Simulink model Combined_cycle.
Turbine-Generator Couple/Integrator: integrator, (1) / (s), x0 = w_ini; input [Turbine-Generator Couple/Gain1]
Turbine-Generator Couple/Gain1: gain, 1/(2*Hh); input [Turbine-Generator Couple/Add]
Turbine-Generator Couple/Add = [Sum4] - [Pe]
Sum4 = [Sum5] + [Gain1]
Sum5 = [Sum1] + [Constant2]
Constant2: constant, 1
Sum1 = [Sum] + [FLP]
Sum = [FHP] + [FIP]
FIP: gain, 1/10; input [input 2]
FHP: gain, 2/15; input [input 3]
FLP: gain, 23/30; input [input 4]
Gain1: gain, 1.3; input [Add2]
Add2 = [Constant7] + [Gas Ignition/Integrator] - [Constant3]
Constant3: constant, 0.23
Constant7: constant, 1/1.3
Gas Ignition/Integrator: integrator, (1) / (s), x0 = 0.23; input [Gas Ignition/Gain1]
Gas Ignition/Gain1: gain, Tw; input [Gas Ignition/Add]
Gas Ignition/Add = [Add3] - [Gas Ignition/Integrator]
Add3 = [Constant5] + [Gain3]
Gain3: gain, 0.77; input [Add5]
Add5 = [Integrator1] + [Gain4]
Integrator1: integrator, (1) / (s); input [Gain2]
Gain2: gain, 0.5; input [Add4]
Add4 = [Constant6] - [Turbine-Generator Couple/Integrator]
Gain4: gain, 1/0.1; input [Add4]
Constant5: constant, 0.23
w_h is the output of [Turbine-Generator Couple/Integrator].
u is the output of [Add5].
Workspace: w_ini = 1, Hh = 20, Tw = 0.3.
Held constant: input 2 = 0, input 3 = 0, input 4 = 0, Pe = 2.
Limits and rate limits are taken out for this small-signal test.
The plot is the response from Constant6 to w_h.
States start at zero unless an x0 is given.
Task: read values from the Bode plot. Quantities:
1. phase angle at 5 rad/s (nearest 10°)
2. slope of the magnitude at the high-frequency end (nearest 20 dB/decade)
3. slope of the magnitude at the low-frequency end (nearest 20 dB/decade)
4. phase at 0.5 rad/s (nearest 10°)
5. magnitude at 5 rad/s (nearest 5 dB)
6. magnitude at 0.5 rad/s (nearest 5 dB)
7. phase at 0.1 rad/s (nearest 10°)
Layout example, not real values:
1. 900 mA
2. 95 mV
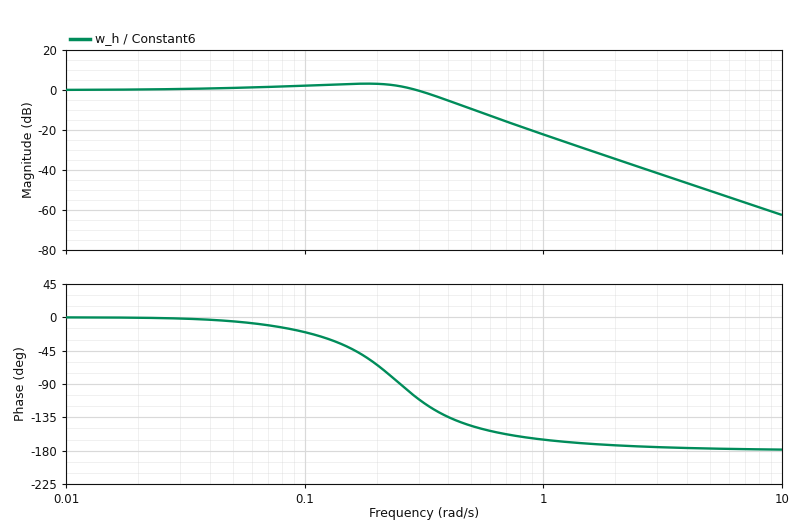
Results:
1. -180°
2. -40 dB/decade
3. 0 dB/decade
4. -150°
5. -50 dB
6. -10 dB
7. -20°
